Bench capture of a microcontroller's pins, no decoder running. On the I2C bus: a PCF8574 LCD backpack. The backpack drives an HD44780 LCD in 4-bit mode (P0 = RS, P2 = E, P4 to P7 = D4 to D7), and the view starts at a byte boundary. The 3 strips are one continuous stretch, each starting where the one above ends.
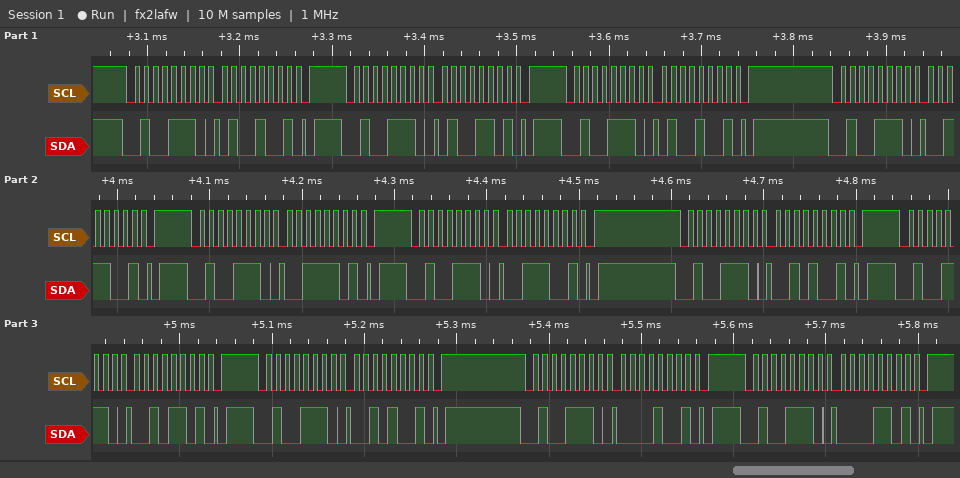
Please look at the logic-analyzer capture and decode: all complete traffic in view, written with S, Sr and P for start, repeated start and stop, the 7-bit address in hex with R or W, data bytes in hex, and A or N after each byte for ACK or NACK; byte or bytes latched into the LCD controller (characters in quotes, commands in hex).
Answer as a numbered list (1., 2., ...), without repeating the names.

1. S 27W A 49 A P S 27W A 4D A P S 27W A 49 A P S 27W A 39 A P S 27W A 3D A P S 27W A 39 A P S 27W A 29 A P S 27W A 2D A P S 27W A 29 A P S 27W A 09 A P S 27W A 0D A P
2. 'C'
